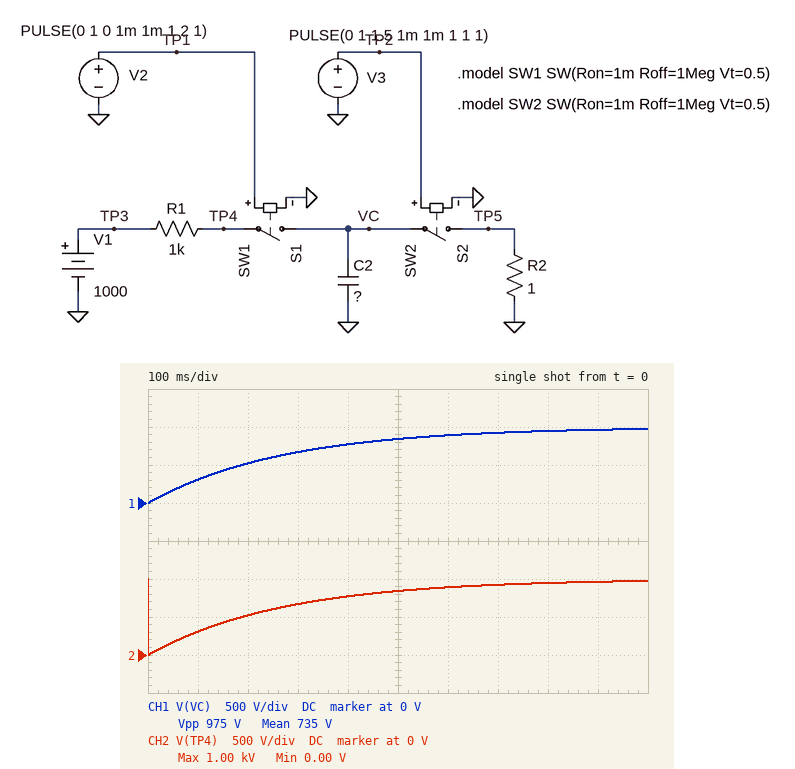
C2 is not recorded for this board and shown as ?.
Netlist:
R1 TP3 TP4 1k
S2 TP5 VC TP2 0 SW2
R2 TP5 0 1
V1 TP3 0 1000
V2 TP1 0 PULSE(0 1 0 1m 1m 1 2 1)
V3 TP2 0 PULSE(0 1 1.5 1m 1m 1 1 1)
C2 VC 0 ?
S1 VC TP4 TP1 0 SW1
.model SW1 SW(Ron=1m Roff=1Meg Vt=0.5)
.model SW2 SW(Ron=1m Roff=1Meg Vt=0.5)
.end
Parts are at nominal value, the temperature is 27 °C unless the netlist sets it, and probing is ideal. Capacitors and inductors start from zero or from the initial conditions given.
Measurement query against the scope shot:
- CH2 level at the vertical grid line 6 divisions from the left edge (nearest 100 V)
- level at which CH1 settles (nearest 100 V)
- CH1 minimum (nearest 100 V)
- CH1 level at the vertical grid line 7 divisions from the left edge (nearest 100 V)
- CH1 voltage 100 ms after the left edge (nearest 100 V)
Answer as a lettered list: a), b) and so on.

a) 900 V
b) 1.0 kV
c) 0 V
d) 900 V
e) 300 V
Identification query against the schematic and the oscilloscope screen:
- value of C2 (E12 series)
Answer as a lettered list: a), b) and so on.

a) 270 µF
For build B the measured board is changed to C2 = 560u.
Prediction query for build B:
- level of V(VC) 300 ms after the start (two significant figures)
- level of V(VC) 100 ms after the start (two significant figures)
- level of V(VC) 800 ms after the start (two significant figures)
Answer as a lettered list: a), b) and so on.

a) 410 V
b) 160 V
c) 760 V
